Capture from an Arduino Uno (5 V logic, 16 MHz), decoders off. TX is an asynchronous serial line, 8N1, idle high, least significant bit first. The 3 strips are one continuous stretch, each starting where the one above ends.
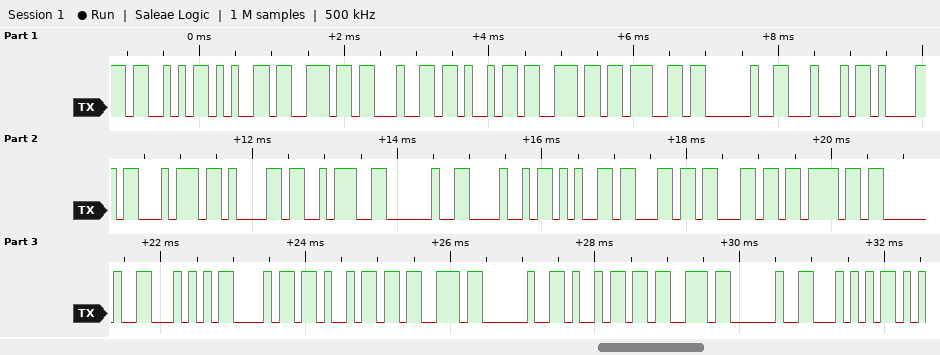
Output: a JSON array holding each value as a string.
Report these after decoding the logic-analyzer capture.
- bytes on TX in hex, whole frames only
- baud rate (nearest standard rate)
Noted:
["53 65 6E 64 69 6E 67 20 44 61 74 61 3A 20 48 65 6C 6C 6F 20 54 68 69 73 20 69 73 20 54", "9600 baud"]
